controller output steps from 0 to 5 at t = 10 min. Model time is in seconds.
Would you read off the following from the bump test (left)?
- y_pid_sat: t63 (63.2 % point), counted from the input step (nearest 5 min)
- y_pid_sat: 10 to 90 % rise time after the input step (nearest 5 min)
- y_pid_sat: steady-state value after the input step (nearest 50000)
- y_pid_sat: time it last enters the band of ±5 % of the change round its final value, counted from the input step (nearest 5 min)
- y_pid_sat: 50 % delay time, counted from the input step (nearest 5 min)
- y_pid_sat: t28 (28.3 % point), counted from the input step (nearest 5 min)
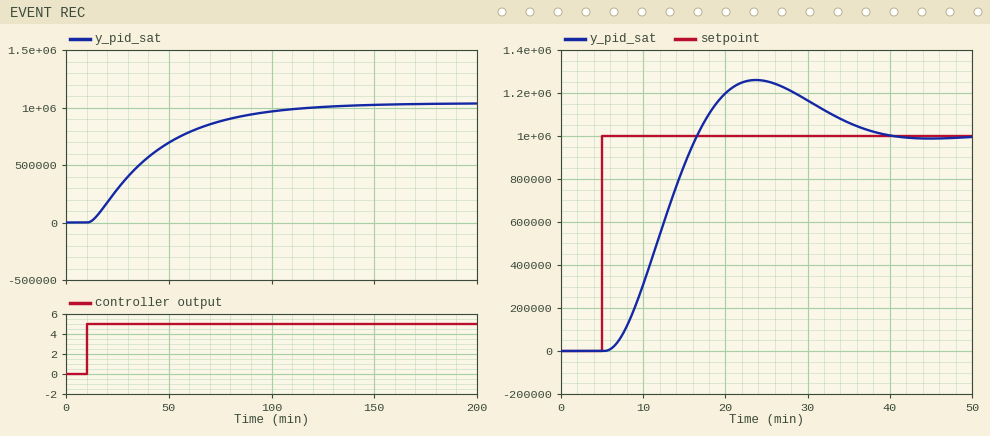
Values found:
35 min
70 min
1050000
100 min
25 min
15 min
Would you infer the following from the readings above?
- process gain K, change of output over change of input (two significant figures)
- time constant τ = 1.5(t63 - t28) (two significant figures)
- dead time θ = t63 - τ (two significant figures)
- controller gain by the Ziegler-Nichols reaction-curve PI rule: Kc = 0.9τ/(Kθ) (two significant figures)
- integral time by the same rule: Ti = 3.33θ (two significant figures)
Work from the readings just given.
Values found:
210000
30 min
5.0 min
0.000026
17 min
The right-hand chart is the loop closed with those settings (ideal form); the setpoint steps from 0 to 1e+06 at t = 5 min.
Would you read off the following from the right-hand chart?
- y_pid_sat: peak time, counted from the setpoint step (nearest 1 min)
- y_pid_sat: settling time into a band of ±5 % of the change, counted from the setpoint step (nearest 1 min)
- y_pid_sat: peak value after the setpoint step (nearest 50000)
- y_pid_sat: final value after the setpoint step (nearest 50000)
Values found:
19 min
31 min
1250000
1000000
